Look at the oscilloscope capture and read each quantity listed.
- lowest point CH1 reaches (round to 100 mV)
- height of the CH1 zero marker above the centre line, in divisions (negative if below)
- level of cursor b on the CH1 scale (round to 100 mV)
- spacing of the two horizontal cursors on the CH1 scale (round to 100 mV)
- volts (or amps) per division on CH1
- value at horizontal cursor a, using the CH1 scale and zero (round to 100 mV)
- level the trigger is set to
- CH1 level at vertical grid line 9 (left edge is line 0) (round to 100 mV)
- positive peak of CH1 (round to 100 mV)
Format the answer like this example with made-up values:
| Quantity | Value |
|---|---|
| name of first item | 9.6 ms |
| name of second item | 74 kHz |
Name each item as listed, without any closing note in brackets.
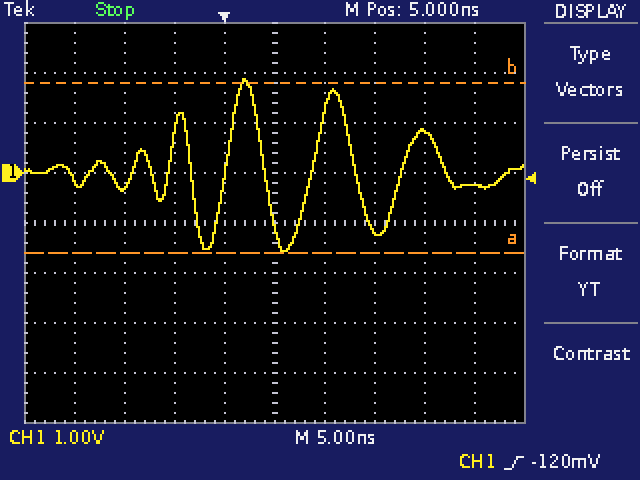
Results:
| Quantity | Value |
|---|---|
| lowest point CH1 reaches | -1.6 V |
| height of the CH1 zero marker above the centre line, in divisions | +1.0 div |
| level of cursor b on the CH1 scale | 1.8 V |
| spacing of the two horizontal cursors on the CH1 scale | 3.4 V |
| volts (or amps) per division on CH1 | 1 V |
| value at horizontal cursor a, using the CH1 scale and zero | -1.6 V |
| level the trigger is set to | -120 mV |
| CH1 level at vertical grid line 9 (left edge is line 0) | -200 mV |
| positive peak of CH1 | 1.9 V |
